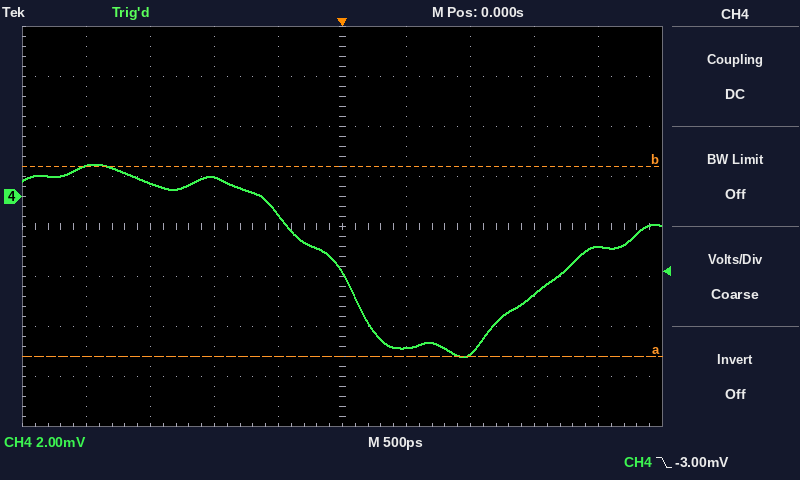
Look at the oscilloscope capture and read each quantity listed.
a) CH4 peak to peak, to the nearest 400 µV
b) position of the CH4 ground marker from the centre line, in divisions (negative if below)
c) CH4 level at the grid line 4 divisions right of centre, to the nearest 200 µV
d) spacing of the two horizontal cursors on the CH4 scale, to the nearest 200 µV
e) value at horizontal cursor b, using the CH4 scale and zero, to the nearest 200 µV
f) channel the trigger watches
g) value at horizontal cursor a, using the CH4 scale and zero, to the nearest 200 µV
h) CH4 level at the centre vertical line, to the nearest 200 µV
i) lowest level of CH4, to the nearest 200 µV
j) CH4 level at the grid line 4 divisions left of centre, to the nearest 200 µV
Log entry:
7.6 mV
+0.6 div
-2.0 mV
7.6 mV
1.2 mV
CH4
-6.4 mV
-3.0 mV
-6.4 mV
1.2 mV
